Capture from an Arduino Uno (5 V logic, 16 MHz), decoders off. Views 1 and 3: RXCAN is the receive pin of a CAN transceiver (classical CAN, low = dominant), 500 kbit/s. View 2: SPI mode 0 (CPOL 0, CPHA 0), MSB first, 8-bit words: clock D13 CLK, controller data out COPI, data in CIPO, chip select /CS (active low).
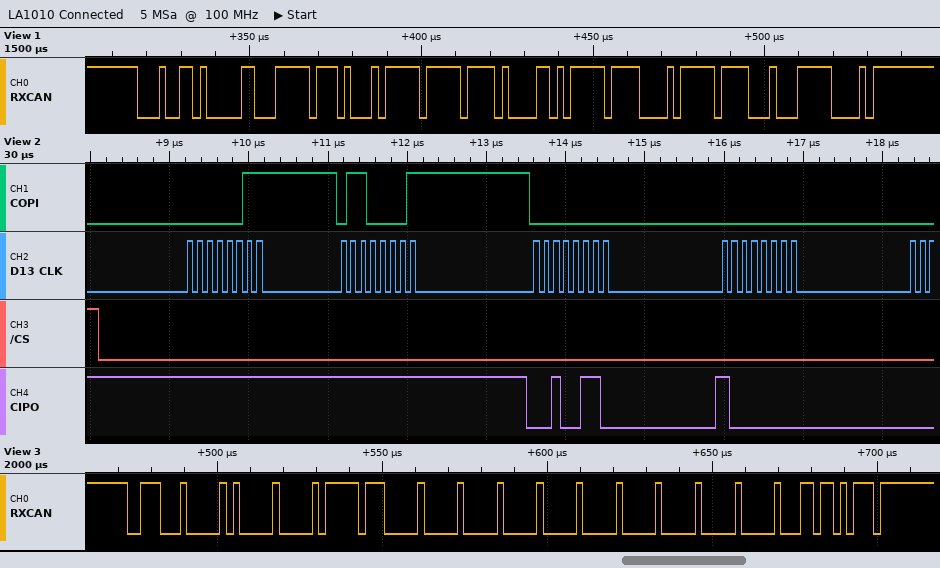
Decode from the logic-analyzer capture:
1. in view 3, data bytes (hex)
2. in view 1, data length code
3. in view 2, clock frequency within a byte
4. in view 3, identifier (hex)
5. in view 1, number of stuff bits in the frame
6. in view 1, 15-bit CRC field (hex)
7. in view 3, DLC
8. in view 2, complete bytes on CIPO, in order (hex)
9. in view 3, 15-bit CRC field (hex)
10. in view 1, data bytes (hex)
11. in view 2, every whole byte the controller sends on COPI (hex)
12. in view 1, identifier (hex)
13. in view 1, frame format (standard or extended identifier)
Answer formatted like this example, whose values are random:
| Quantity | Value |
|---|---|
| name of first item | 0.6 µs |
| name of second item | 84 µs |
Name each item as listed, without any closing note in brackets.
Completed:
| Quantity | Value |
|---|---|
| in view 3, data bytes | 00 FF 00 00 00 00 00 00 |
| in view 1, data length code | 8 |
| in view 2, clock frequency within a byte | 8 MHz |
| in view 3, identifier | 0x388 |
| in view 1, number of stuff bits in the frame | 7 |
| in view 1, 15-bit CRC field | 0x08F8 |
| in view 3, DLC | 8 |
| in view 2, complete bytes on CIPO, in order | FF FF 26 80 |
| in view 3, 15-bit CRC field | 0x036B |
| in view 1, data bytes | FF 45 FF FA 1A FF 85 FF |
| in view 2, every whole byte the controller sends on COPI | 03 61 00 00 |
| in view 1, identifier | 0x134 |
| in view 1, frame format | standard |
